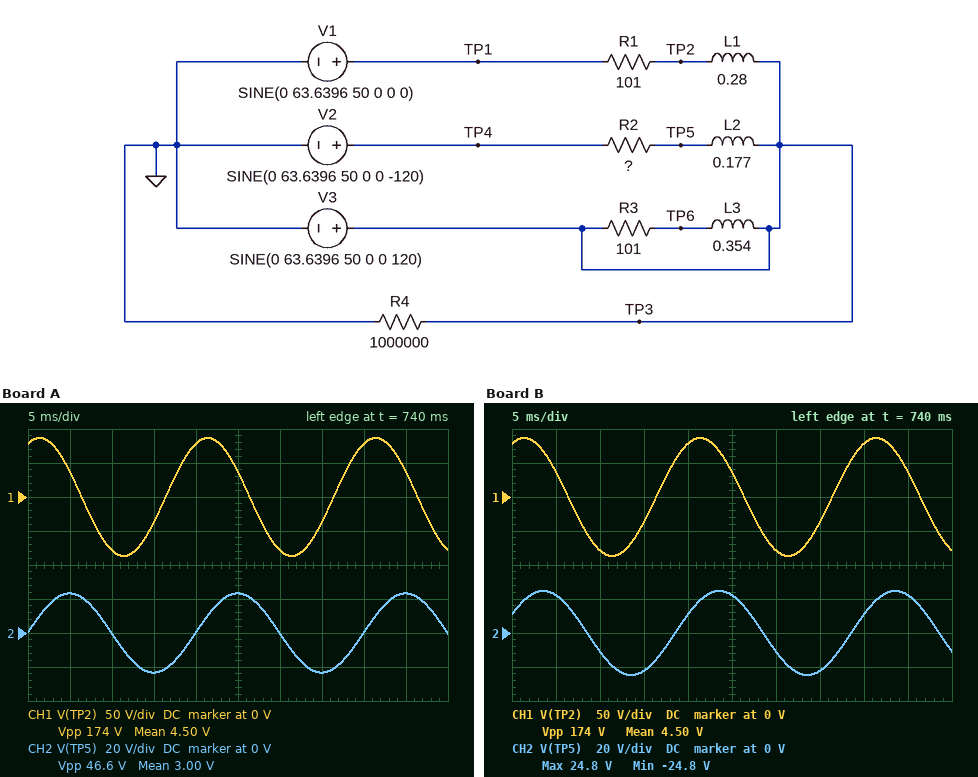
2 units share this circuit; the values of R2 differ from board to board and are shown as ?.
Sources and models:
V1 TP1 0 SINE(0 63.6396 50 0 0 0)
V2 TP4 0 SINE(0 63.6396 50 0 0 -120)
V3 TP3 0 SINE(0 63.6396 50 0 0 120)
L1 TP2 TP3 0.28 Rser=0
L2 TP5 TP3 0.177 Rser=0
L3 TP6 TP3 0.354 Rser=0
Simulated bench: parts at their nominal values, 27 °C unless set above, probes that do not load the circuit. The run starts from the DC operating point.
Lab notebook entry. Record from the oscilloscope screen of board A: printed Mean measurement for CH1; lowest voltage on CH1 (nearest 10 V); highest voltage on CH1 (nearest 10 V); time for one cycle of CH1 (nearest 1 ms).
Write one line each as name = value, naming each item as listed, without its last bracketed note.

printed Mean measurement for CH1 = 4.50 V
lowest voltage on CH1 = -90 V
highest voltage on CH1 = 90 V
time for one cycle of CH1 = 20 ms
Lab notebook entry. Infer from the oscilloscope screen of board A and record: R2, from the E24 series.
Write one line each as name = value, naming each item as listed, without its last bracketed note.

R2, from the E24 series = 56 Ω
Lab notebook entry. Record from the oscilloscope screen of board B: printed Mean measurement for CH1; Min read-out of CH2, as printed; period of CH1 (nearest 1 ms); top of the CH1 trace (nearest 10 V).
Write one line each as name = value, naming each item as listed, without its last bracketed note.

printed Mean measurement for CH1 = 4.50 V
Min read-out of CH2, as printed = -24.8 V
period of CH1 = 20 ms
top of the CH1 trace = 90 V
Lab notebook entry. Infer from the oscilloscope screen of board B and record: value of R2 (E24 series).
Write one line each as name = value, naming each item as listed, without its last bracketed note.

value of R2 = 68 Ω
